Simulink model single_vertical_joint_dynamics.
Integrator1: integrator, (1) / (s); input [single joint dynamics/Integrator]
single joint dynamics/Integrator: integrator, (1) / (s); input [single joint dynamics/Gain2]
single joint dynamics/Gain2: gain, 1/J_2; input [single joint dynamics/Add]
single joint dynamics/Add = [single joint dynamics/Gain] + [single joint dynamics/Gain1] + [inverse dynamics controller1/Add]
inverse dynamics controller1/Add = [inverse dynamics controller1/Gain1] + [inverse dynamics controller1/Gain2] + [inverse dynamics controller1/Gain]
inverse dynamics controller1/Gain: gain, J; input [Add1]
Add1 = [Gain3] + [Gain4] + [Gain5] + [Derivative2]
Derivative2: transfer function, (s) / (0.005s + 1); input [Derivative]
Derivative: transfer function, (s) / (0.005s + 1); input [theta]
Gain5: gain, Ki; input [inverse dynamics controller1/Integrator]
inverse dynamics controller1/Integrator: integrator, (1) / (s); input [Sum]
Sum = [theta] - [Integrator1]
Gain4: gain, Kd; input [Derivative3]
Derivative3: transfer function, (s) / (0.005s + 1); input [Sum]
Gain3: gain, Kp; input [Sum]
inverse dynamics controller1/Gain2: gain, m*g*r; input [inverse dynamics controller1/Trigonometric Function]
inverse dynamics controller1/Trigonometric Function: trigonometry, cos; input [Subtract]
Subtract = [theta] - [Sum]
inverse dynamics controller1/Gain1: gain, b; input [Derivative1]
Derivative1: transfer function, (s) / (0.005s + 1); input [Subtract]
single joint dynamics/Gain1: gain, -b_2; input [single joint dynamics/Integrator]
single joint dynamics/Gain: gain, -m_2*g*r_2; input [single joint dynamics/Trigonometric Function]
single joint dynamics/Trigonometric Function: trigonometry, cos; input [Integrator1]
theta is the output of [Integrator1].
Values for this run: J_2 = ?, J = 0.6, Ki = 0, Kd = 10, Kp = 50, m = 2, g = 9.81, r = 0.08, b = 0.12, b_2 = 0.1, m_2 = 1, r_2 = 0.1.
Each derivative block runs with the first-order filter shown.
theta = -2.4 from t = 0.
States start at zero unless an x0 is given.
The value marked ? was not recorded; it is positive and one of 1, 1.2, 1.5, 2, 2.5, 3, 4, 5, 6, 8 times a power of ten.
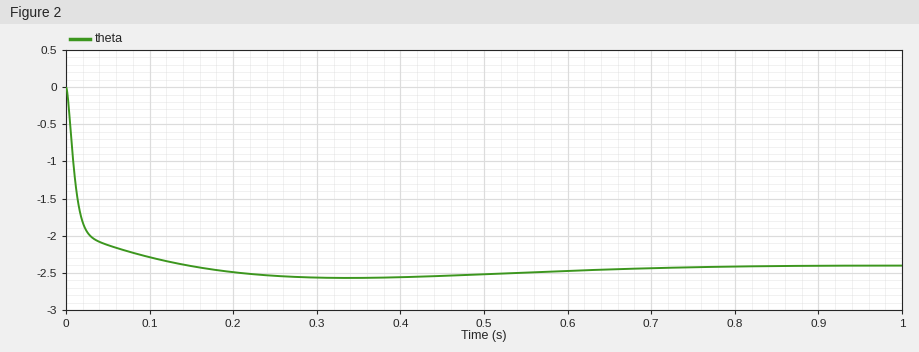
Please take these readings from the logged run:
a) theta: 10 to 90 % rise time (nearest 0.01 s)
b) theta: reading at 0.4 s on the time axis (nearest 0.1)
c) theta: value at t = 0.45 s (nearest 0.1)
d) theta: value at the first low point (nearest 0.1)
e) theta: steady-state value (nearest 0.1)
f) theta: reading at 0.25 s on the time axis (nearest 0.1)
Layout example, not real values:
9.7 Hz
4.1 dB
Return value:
0.06 s
-2.6
-2.5
-2.6
-2.4
-2.5
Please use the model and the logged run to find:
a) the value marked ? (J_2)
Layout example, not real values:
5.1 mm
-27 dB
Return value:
0.8
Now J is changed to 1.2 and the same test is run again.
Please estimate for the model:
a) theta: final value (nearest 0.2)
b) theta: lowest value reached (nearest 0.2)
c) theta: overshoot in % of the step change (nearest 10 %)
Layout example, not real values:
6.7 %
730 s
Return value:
-2.4
-3.6
50 %
